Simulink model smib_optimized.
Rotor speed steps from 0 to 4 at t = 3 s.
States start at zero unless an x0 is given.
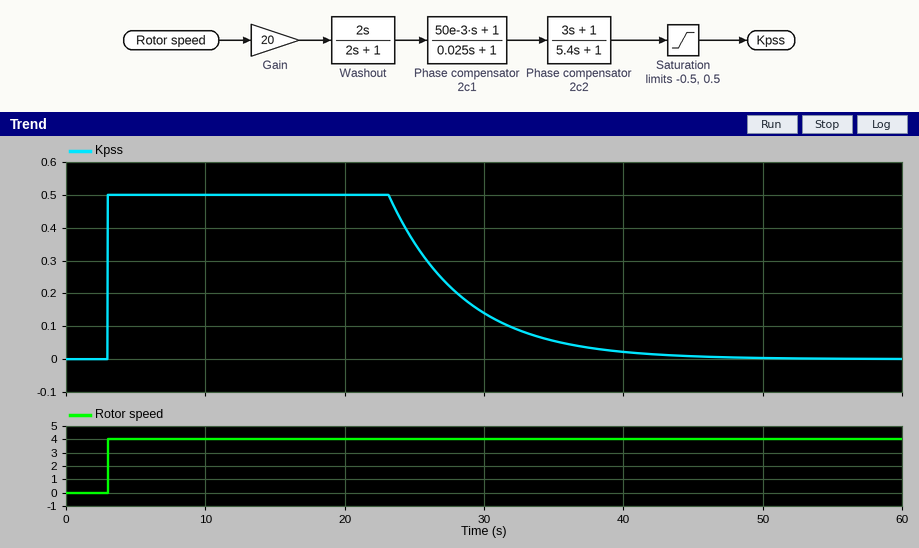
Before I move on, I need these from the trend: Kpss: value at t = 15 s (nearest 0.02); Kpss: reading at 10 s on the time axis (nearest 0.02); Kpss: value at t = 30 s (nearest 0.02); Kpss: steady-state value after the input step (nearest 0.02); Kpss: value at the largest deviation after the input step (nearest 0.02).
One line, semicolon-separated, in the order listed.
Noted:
0.50; 0.50; 0.14; 0.00; 0.50
